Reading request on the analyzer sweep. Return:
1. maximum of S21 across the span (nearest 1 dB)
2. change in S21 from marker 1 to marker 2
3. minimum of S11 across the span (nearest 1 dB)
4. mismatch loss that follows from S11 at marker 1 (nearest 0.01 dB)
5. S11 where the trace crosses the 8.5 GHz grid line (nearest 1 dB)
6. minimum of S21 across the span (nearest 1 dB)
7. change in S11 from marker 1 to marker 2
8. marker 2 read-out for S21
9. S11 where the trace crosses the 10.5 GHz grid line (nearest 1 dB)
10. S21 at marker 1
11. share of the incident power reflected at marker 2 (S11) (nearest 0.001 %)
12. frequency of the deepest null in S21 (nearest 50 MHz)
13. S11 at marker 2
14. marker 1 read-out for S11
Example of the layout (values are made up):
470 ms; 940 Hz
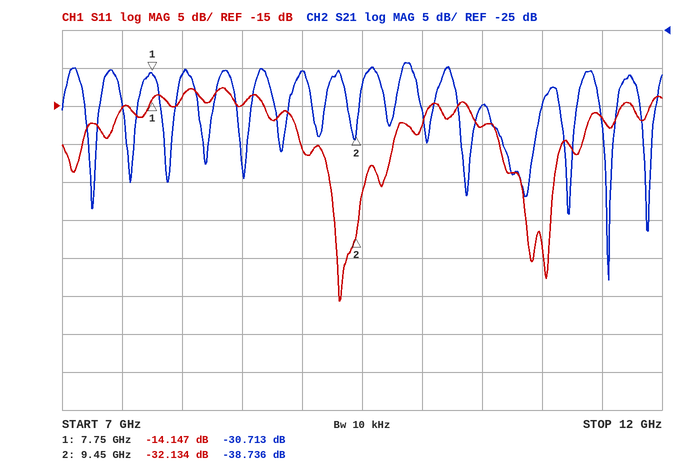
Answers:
-29 dB; -8.023 dB; -41 dB; 0.17 dB; -15 dB; -58 dB; -17.987 dB; -38.736 dB; -18 dB; -30.713 dB; 0.061 %; 11.55 GHz; -32.134 dB; -14.147 dB
